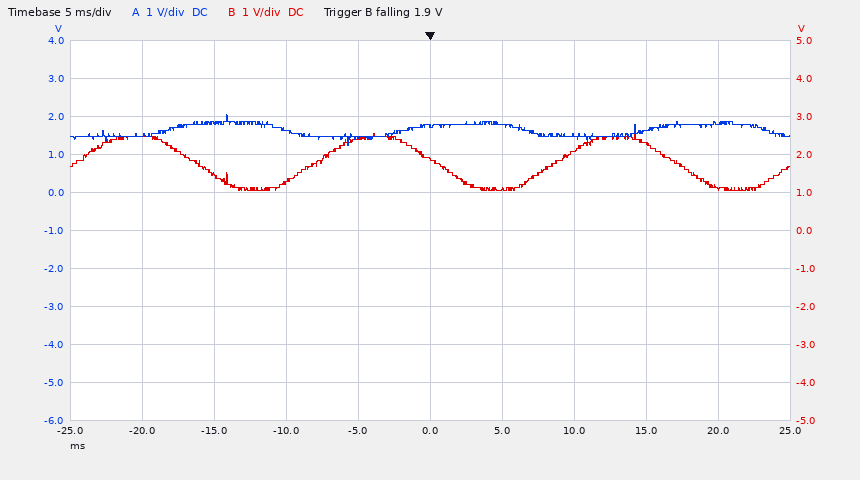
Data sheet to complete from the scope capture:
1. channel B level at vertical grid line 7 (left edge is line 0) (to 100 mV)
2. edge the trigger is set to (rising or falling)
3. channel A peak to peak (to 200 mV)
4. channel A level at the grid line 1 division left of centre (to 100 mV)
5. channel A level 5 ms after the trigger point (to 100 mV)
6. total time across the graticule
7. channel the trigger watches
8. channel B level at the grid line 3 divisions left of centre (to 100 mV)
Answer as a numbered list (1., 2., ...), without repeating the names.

1. 2.1 V
2. falling
3. 800 mV
4. 1.4 V
5. 1.8 V
6. 50 ms
7. channel B
8. 1.4 V
